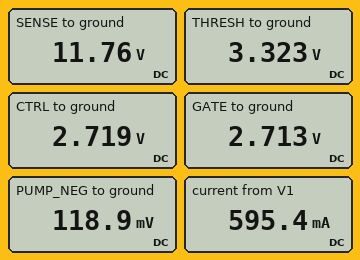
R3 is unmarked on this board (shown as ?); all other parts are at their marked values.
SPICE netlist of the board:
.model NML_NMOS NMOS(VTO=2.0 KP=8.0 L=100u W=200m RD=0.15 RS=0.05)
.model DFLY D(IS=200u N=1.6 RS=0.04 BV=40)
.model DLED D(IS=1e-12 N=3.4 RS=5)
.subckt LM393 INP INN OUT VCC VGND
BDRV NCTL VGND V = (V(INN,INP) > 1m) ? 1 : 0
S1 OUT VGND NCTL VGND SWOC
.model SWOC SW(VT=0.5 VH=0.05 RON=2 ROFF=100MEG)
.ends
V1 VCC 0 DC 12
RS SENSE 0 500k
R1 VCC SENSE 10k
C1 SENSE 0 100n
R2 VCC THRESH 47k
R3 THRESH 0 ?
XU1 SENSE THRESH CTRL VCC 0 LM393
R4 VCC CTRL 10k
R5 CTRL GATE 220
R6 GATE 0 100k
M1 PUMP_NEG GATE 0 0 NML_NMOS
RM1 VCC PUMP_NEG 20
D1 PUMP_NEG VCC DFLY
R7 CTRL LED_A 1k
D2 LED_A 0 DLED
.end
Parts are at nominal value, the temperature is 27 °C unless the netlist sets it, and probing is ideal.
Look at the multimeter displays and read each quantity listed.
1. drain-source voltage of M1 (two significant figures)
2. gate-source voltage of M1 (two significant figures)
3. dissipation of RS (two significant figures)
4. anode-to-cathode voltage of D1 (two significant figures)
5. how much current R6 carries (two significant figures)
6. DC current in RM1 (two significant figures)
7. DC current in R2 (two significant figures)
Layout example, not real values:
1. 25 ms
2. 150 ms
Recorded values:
1. 120 mV
2. 2.7 V
3. 280 µW
4. -12 V
5. 27 µA
6. 590 mA
7. 180 µA
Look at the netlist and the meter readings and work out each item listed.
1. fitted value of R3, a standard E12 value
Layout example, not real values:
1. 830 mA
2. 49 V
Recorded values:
1. 18 kΩ
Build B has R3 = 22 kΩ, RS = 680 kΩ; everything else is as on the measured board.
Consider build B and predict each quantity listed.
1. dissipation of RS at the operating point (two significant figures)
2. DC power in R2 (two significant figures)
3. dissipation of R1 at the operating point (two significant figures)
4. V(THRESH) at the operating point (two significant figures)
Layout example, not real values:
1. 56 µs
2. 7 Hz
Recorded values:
1. 210 µW
2. 1.4 mW
3. 3.0 µW
4. 3.8 V
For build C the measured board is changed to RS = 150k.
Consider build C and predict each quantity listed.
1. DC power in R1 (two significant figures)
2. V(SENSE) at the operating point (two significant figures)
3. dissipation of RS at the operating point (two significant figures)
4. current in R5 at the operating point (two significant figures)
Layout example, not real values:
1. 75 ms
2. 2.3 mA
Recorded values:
1. 56 µW
2. 11 V
3. 840 µW
4. 27 µA
